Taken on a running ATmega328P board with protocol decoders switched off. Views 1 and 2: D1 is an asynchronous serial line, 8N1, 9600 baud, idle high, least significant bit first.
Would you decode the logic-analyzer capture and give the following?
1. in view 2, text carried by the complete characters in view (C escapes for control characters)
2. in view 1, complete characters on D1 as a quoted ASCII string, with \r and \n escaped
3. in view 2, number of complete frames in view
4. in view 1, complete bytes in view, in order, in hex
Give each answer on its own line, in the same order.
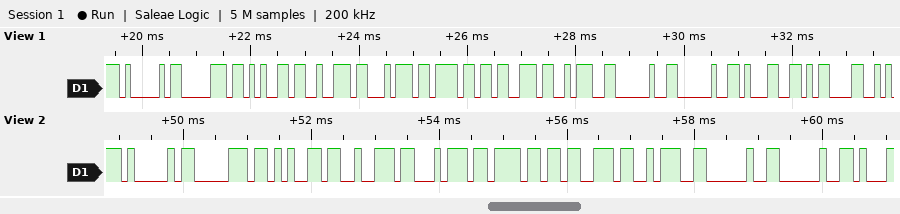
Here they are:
"Apertos:  "
"Apertos:  1\r"
10
41 70 65 72 74 6F 73 3A 20 20 31 0D
